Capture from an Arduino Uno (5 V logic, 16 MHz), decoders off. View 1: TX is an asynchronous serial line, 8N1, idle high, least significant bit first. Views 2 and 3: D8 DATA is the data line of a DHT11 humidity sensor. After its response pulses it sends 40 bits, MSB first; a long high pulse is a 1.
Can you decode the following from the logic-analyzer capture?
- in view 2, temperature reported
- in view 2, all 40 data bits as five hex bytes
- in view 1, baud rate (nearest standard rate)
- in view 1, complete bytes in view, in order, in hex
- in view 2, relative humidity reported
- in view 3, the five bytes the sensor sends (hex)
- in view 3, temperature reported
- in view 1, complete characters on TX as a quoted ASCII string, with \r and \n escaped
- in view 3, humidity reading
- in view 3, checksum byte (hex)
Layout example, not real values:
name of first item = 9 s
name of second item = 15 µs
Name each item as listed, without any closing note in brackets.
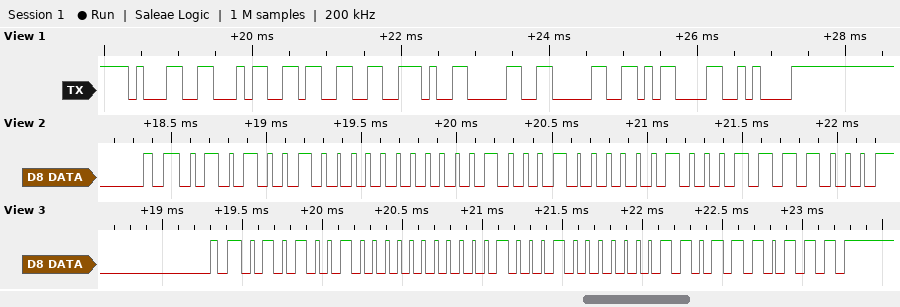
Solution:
in view 2, temperature reported = 34.4 °C
in view 2, all 40 data bits as five hex bytes = 52 00 22 04 78
in view 1, baud rate = 9600 baud
in view 1, complete bytes in view, in order, in hex = 31 34 33 2E 30 30 0D 0A
in view 2, relative humidity reported = 82 %
in view 3, the five bytes the sensor sends = 52 00 22 03 77
in view 3, temperature reported = 34.3 °C
in view 1, complete characters on TX as a quoted ASCII string, with \r and \n escaped = "143.00\r\n"
in view 3, humidity reading = 82 %
in view 3, checksum byte = 0x77
